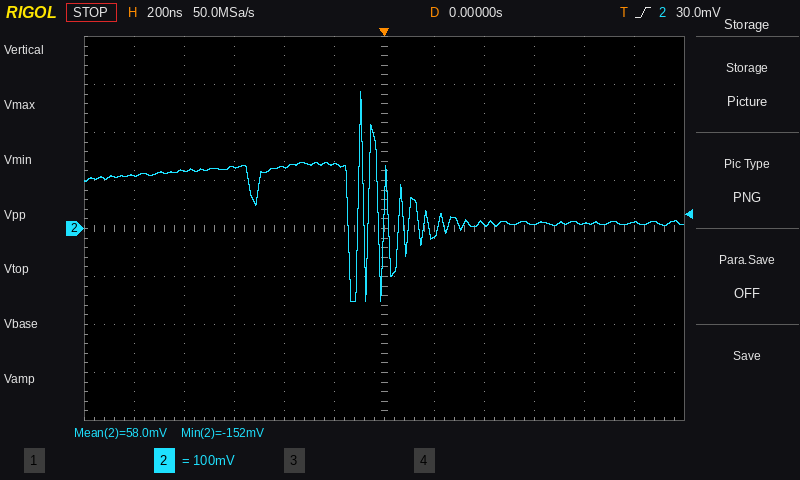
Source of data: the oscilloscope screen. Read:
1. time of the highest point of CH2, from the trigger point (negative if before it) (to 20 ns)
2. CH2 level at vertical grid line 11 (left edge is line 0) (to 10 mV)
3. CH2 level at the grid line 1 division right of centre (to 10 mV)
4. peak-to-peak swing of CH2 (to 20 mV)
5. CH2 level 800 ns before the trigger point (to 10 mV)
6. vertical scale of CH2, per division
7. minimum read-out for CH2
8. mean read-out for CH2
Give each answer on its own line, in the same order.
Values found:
-100 ns
10 mV
-10 mV
440 mV
120 mV
100 mV
-152 mV
58.0 mV
